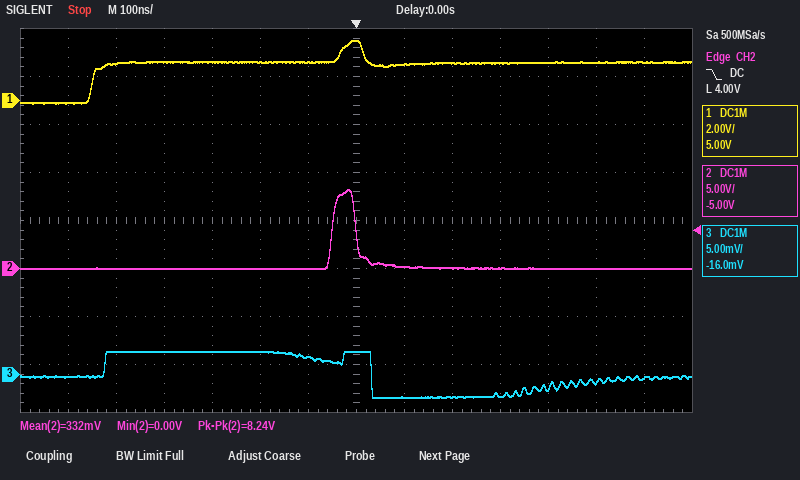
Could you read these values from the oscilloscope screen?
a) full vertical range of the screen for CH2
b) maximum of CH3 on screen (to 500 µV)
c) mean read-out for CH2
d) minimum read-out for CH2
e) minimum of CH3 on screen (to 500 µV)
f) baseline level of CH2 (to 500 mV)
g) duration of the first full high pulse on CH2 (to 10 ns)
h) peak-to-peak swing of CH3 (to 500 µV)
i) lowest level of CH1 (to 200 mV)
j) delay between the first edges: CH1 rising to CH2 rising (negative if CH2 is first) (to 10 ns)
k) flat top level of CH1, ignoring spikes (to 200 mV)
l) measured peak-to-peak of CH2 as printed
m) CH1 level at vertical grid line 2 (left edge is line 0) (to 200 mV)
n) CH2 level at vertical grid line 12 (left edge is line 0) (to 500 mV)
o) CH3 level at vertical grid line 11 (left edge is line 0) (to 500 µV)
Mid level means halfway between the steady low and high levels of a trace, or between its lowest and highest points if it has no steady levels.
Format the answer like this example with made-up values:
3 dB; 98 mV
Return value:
40 V; 2.5 mV; 332 mV; 0.00 V; -2.5 mV; 0.0 V; 50 ns; 5.0 mV; -200 mV; +500 ns; 1.6 V; 8.24 V; 1.6 V; 0.0 V; -1.5 mV
